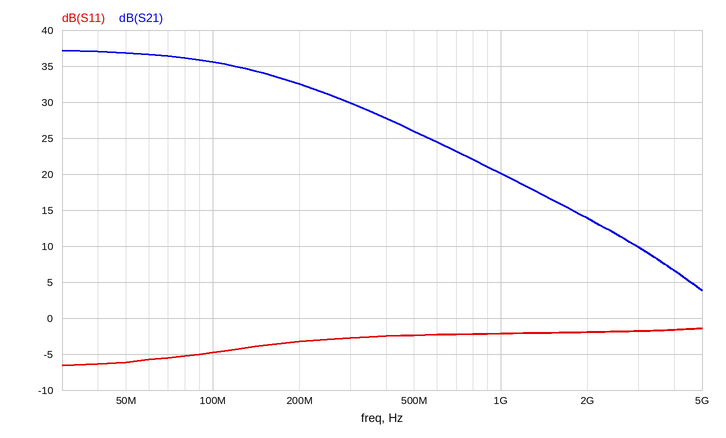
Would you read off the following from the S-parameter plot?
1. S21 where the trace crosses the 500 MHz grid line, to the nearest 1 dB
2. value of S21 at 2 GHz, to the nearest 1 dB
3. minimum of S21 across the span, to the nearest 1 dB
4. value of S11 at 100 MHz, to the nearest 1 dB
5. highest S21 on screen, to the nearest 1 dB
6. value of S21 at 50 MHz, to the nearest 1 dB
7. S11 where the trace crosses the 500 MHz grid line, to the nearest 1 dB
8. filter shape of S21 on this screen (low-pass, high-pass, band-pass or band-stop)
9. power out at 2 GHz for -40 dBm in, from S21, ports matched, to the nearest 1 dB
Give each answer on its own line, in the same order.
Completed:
26 dB
14 dB
4 dB
-5 dB
37 dB
37 dB
-2 dB
low-pass
-26 dBm
